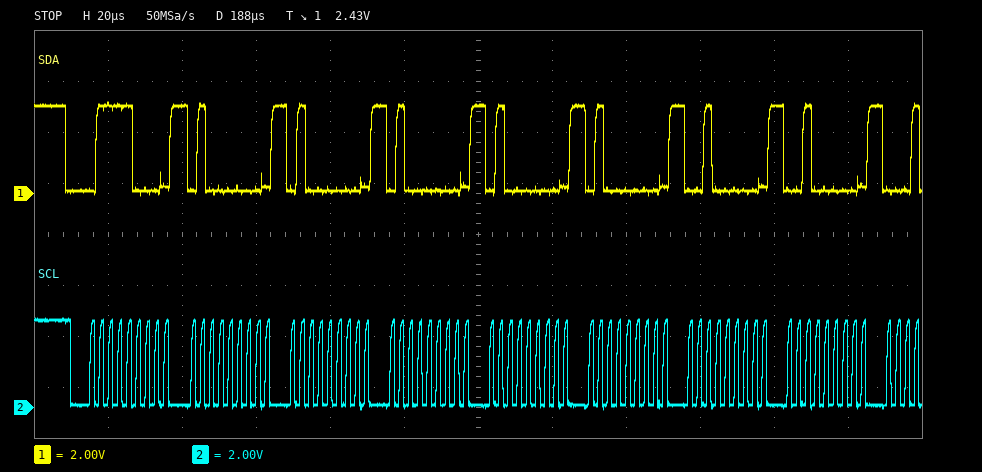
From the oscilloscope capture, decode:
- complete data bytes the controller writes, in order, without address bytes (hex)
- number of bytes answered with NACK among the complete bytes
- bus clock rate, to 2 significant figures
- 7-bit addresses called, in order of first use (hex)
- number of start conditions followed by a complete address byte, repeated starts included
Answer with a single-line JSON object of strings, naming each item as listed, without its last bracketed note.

{"complete data bytes the controller writes, in order, without address bytes": "40 40 40 40 40 20 20", "number of bytes answered with NACK among the complete bytes": "0", "bus clock rate, to 2 significant figures": "400 kHz", "7-bit addresses called, in order of first use": "0x3C", "number of start conditions followed by a complete address byte, repeated starts included": "1"}
